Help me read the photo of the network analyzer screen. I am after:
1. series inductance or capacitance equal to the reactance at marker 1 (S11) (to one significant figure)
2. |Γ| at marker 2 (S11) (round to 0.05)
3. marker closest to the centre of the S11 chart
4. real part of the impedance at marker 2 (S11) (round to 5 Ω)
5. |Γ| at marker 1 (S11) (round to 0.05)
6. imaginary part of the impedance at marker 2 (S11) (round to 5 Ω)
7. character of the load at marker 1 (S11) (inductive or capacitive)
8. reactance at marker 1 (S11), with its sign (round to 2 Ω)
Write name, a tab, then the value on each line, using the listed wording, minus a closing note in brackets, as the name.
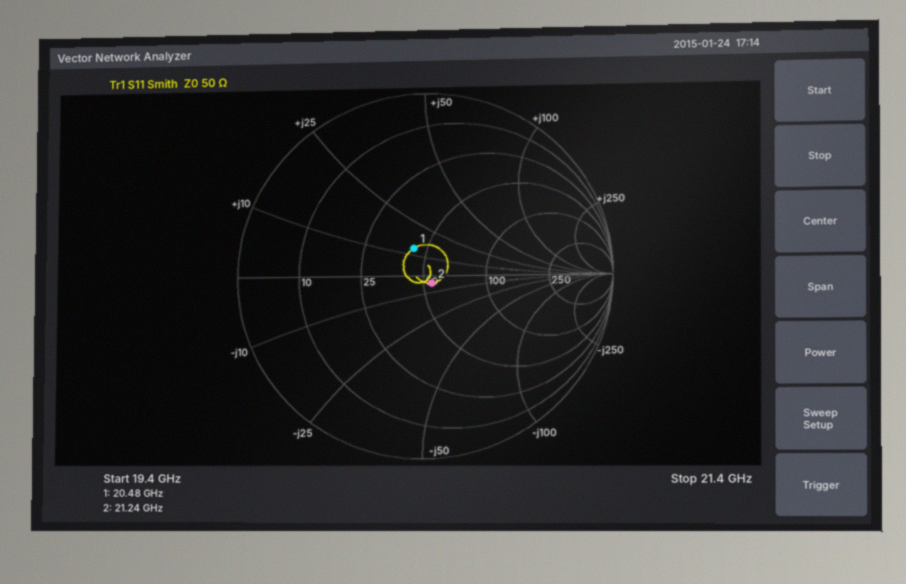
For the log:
series inductance or capacitance equal to the reactance at marker 1 (S11)	100 pH
|Γ| at marker 2 (S11)	0.05
marker closest to the centre of the S11 chart	marker 2
real part of the impedance at marker 2 (S11)	55 Ω
|Γ| at marker 1 (S11)	0.15
imaginary part of the impedance at marker 2 (S11)	-5 Ω
character of the load at marker 1 (S11)	inductive
reactance at marker 1 (S11), with its sign	+14 Ω
